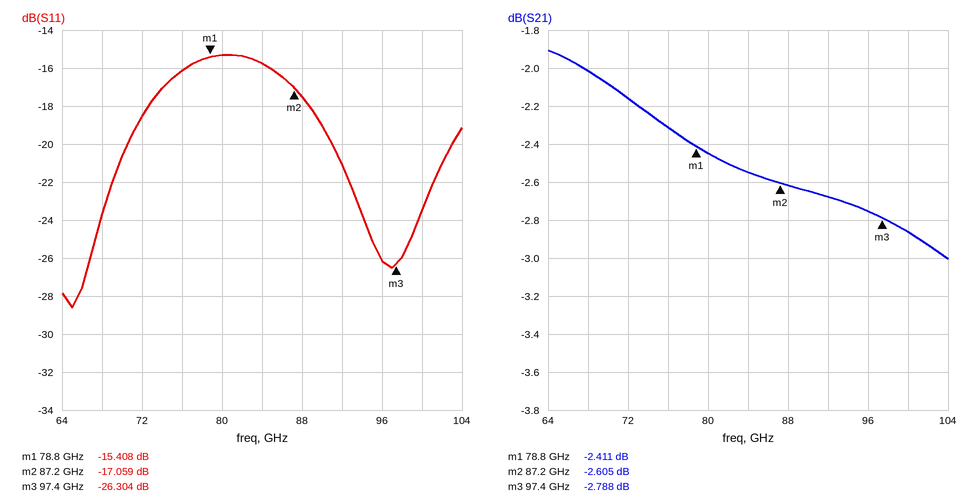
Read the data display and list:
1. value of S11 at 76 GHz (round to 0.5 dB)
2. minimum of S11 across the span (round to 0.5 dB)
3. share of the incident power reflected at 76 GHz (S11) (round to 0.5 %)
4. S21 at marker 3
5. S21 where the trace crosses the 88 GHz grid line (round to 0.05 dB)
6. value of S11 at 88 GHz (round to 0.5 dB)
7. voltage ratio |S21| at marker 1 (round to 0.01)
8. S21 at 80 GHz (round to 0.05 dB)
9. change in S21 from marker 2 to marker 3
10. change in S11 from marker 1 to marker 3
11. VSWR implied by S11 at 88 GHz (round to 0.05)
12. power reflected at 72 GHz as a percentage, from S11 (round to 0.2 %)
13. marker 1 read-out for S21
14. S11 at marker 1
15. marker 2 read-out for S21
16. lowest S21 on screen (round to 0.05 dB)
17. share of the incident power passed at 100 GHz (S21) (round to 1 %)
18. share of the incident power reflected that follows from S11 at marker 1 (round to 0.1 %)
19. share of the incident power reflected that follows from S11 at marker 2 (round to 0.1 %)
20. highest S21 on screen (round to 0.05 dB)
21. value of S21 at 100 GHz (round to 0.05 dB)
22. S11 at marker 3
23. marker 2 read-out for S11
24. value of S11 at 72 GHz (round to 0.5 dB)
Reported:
-16.0 dB
-28.5 dB
2.5 %
-2.788 dB
-2.60 dB
-17.5 dB
0.76
-2.45 dB
-0.183 dB
-10.896 dB
1.30
1.4 %
-2.411 dB
-15.408 dB
-2.605 dB
-3.00 dB
52 %
2.9 %
2.0 %
-1.90 dB
-2.85 dB
-26.304 dB
-17.059 dB
-18.5 dB
